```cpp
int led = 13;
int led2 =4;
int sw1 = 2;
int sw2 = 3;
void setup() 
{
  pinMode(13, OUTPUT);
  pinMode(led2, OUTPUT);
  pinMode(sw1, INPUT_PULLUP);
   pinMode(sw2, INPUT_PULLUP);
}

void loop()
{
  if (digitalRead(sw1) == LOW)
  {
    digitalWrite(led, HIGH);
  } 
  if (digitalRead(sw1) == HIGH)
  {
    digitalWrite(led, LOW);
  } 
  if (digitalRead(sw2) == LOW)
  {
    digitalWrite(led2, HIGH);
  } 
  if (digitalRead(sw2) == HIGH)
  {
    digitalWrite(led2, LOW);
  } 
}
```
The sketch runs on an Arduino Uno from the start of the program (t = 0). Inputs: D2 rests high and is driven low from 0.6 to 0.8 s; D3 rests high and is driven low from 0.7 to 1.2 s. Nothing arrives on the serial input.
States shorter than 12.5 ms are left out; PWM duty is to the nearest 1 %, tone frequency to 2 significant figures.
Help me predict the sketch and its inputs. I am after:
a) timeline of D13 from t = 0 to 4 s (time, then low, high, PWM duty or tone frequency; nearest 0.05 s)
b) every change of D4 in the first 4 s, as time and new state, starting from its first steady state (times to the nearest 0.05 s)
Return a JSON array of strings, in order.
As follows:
["0 s low; 0.6 s high; 0.8 s low", "0 s low; 0.7 s high; 1.2 s low"]
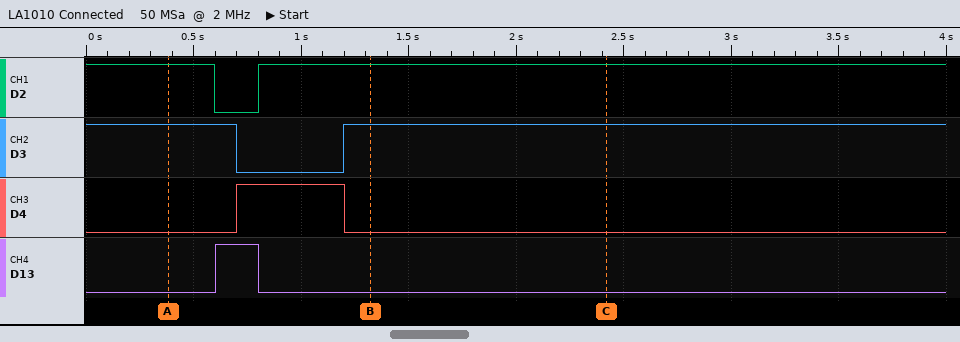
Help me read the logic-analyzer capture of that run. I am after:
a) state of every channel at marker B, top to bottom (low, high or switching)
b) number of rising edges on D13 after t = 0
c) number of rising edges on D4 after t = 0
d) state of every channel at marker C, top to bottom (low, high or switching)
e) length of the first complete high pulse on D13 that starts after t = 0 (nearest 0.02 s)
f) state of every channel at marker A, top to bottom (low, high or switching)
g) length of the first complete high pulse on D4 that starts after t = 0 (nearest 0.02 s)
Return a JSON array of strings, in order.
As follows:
["D2 high, D3 high, D4 low, D13 low", "1", "1", "D2 high, D3 high, D4 low, D13 low", "0.20 s", "D2 high, D3 high, D4 low, D13 low", "0.50 s"]
